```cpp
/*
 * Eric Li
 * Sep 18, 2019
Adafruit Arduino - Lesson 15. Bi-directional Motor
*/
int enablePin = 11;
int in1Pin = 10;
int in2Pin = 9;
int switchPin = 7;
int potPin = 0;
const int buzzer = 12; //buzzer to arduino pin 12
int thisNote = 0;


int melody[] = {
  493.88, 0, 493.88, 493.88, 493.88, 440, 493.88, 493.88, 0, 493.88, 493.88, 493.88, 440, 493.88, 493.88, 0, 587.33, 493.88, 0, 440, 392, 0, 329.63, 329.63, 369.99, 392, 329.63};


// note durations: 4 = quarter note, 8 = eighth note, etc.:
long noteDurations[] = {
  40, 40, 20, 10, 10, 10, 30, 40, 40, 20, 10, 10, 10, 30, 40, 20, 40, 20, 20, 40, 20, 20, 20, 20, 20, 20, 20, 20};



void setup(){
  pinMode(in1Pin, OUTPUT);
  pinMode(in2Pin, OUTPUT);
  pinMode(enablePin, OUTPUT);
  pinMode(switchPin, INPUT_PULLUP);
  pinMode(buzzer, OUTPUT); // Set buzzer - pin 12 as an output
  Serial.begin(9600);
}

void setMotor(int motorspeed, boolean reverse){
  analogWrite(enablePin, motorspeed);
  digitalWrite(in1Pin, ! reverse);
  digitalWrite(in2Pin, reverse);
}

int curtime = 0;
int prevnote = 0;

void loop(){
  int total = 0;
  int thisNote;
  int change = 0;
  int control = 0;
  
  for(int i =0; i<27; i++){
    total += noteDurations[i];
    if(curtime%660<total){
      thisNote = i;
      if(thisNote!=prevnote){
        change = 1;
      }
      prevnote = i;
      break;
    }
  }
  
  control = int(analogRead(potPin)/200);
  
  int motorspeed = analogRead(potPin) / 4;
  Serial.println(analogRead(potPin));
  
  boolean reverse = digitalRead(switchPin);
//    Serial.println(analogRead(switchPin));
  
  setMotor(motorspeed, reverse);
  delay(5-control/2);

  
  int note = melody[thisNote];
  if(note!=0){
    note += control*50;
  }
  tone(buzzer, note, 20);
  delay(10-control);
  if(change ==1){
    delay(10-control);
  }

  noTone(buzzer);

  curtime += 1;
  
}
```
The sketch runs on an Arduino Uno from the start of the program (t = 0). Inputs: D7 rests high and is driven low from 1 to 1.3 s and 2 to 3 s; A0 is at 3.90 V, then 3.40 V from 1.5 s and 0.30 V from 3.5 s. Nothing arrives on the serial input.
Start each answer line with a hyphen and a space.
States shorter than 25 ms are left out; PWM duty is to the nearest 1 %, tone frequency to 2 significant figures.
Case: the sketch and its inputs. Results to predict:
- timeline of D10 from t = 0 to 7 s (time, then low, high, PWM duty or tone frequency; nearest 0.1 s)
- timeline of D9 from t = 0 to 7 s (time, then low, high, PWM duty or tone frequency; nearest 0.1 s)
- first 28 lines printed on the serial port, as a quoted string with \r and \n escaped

- 0 s low; 1 s high; 1.3 s low; 2 s high; 3 s low
- 0 s high; 1 s low; 1.3 s high; 2 s low; 3 s high
- "798\r\n798\r\n798\r\n798\r\n798\r\n798\r\n798\r\n798\r\n798\r\n798\r\n798\r\n798\r\n798\r\n798\r\n798\r\n798\r\n798\r\n798\r\n798\r\n798\r\n798\r\n798\r\n798\r\n798\r\n798\r\n798\r\n798\r\n798\r\n"
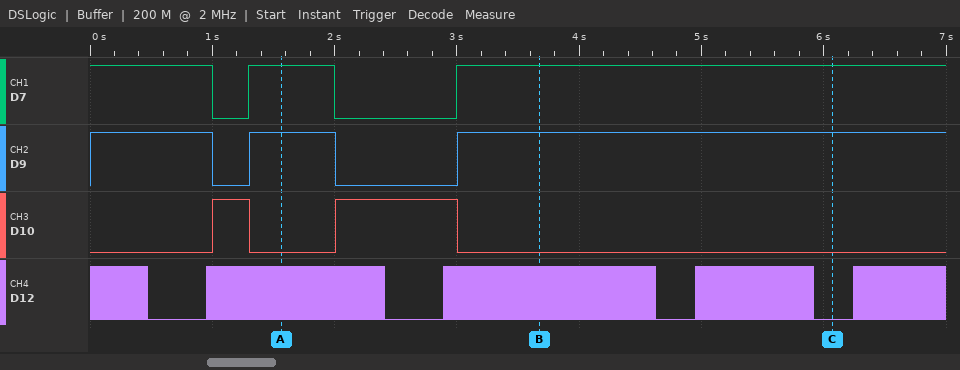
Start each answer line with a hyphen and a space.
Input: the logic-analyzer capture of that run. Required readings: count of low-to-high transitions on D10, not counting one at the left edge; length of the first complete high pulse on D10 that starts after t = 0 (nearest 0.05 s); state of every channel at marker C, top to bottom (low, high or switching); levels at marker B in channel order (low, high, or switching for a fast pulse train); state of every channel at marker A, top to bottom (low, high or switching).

- 2
- 0.30 s
- D7 high, D9 high, D10 low, D12 low
- D7 high, D9 high, D10 low, D12 switching
- D7 high, D9 high, D10 low, D12 switching
